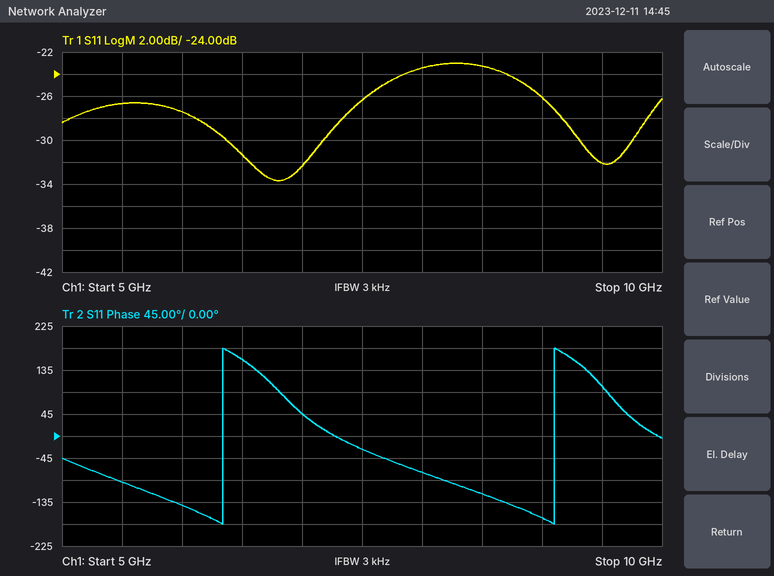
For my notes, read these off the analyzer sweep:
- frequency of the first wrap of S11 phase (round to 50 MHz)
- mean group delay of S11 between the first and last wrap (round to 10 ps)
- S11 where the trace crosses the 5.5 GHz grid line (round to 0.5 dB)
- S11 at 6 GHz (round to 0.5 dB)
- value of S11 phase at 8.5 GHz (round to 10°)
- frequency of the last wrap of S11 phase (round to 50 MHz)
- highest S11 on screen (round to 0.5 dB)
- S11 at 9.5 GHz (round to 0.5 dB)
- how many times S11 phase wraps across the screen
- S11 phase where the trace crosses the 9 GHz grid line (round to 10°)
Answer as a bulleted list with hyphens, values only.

- 6.35 GHz
- 360 ps
- -26.5 dB
- -27.5 dB
- -120°
- 9.10 GHz
- -23.0 dB
- -32.0 dB
- 2
- -170°
